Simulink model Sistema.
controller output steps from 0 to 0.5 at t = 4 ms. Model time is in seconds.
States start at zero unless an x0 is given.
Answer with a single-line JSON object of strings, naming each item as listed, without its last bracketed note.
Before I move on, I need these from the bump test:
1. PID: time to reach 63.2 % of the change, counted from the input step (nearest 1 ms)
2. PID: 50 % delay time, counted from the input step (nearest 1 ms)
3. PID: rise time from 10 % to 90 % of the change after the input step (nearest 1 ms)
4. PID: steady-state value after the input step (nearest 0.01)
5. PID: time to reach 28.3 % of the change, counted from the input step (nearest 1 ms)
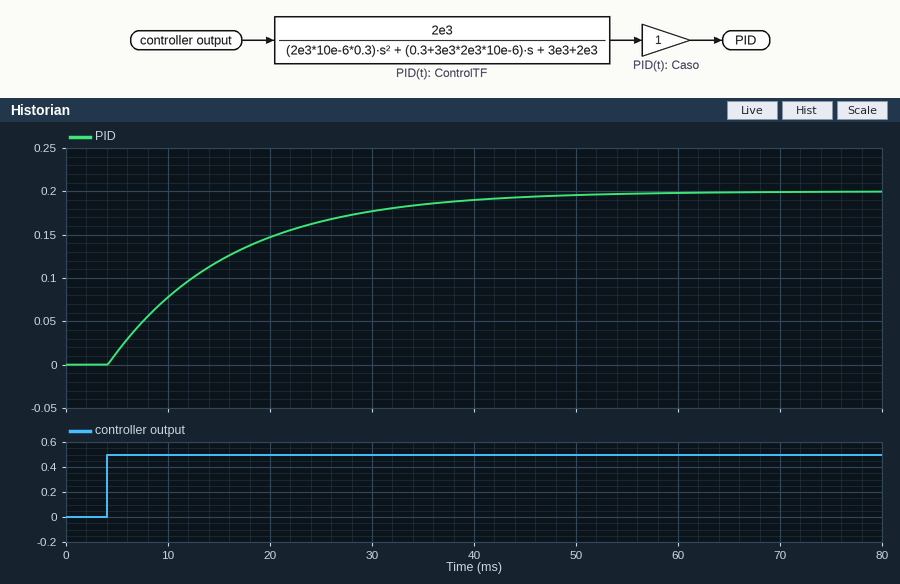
{"PID: time to reach 63.2 % of the change, counted from the input step": "12 ms", "PID: 50 % delay time, counted from the input step": "8 ms", "PID: rise time from 10 % to 90 % of the change after the input step": "26 ms", "PID: steady-state value after the input step": "0.20", "PID: time to reach 28.3 % of the change, counted from the input step": "4 ms"}
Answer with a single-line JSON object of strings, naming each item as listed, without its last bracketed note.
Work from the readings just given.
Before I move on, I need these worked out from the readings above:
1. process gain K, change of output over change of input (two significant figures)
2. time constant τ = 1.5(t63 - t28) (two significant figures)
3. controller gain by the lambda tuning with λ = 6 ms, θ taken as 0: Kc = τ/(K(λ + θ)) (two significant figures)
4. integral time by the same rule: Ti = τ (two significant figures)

{"process gain K, change of output over change of input": "0.40", "time constant τ = 1.5(t63 - t28)": "12 ms", "controller gain by the lambda tuning with λ = 6 ms, θ taken as 0: Kc = τ/(K(λ + θ))": "5.0", "integral time by the same rule: Ti = τ": "12 ms"}
